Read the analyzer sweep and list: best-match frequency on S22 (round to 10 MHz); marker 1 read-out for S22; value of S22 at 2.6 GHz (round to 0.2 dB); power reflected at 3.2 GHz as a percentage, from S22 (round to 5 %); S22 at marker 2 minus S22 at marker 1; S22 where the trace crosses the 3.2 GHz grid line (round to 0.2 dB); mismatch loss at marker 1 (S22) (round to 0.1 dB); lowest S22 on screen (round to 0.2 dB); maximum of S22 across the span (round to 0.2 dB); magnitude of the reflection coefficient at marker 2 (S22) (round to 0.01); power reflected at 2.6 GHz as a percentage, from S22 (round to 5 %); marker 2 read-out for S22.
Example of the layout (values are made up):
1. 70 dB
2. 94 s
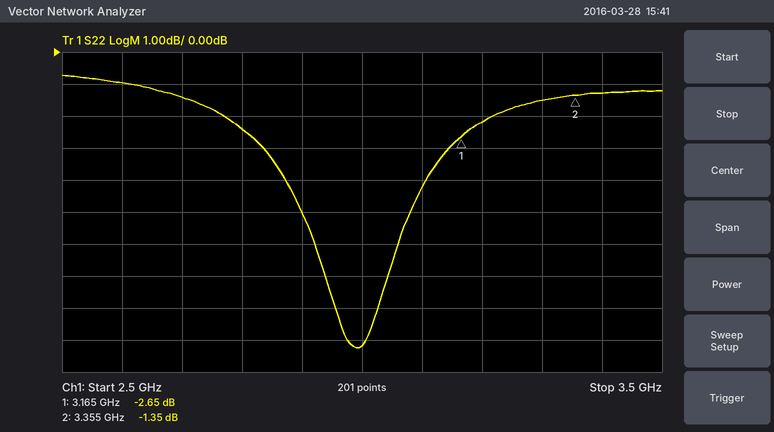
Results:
1. 2.99 GHz
2. -2.65 dB
3. -1.0 dB
4. 60 %
5. 1.30 dB
6. -2.2 dB
7. 3.4 dB
8. -9.2 dB
9. -0.8 dB
10. 0.86
11. 80 %
12. -1.35 dB
